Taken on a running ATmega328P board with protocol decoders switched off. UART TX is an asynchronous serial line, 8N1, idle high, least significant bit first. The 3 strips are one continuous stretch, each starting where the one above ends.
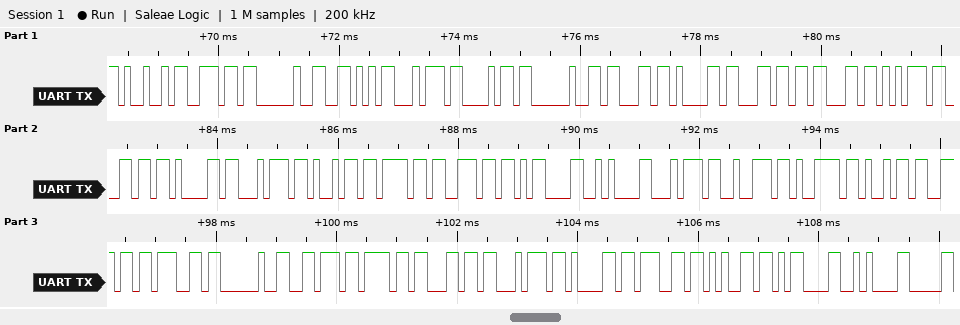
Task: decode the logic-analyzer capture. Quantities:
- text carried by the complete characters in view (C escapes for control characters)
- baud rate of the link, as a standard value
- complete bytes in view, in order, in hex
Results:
"In Vth calculation\r\ntrying voltage\r\n"
9600 baud
49 6E 20 56 74 68 20 63 61 6C 63 75 6C 61 74 69 6F 6E 0D 0A 74 72 79 69 6E 67 20 76 6F 6C 74 61 67 65 0D 0A
